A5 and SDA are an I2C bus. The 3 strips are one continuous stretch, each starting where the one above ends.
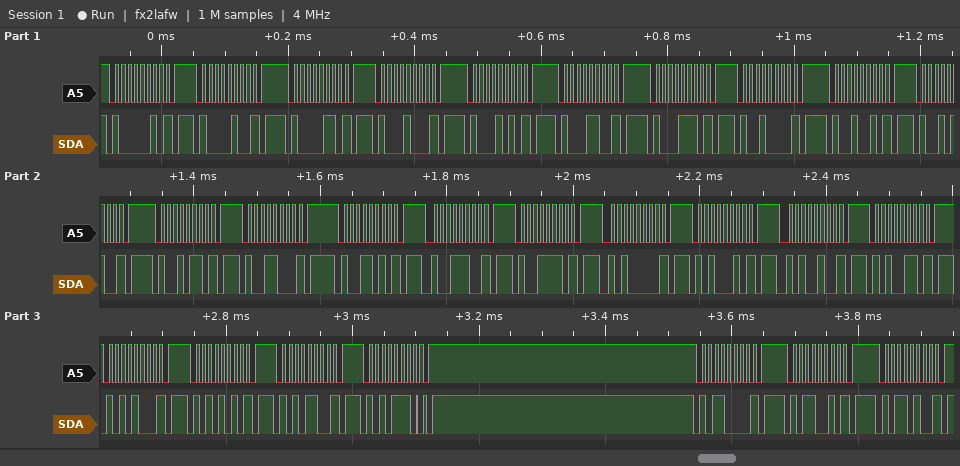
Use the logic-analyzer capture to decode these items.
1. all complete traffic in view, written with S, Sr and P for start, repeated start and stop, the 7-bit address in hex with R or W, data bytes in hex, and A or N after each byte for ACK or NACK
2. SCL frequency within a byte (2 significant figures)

S 41W N P S 42W N P S 43W N P S 44W N P S 45W N P S 46W N P S 47W N P S 48W N P S 49W N P S 4AW N P S 4BW N P S 4CW N P S 4DW N P S 4EW N P S 4FW N P S 50W N P S 51W N P S 52W N P S 53W N P S 54W N P S 55W N P S 56W N P S 57W A P S 58W N P S 59W N P S 5AW N P
100 kHz
